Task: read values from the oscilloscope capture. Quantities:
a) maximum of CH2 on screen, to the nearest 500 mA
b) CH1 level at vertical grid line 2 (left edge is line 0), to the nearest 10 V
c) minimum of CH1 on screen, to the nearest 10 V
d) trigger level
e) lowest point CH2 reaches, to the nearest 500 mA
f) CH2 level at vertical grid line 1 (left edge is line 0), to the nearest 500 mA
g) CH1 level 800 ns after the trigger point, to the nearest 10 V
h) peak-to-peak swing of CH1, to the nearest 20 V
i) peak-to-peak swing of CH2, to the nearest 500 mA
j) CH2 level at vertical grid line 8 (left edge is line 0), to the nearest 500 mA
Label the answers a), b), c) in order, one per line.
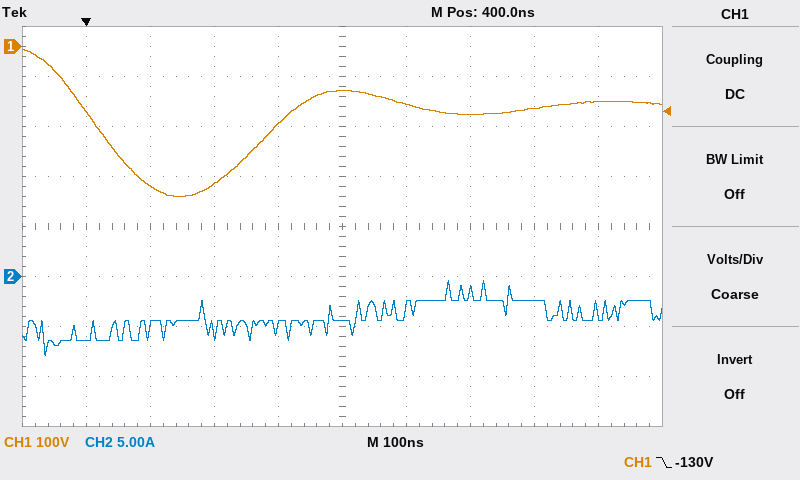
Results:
a) -500 mA
b) -280 V
c) -300 V
d) -130 V
e) -8.0 A
f) -6.5 A
g) -110 V
h) 300 V
i) 7.5 A
j) -2.5 A
